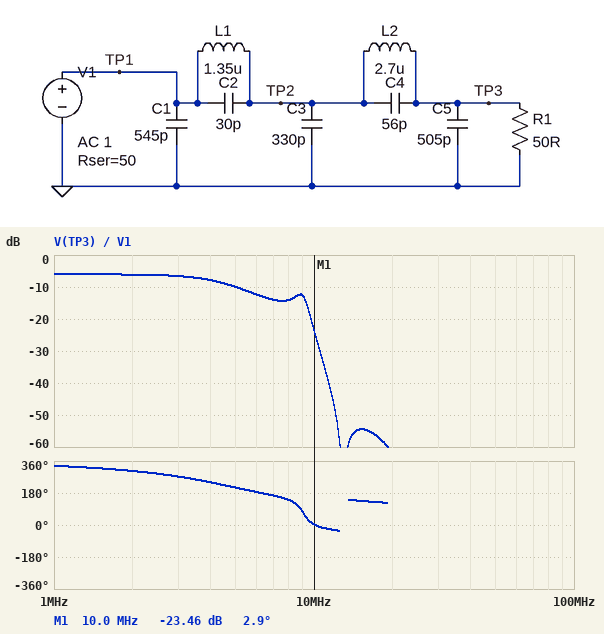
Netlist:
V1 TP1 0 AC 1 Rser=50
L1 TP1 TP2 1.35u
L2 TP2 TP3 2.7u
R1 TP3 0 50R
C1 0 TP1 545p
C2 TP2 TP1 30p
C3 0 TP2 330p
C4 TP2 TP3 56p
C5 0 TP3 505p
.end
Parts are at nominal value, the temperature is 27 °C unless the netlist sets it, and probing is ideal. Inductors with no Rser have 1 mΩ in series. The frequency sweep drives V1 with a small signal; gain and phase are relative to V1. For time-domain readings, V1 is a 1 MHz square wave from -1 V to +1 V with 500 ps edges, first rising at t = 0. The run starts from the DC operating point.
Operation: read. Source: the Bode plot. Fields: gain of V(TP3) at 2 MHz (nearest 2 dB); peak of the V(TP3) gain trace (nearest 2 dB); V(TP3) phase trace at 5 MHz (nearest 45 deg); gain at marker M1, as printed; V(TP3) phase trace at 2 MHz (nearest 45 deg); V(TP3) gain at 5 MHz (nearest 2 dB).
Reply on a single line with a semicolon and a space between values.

-6 dB; -6 dB; 225 deg; -23.46 dB; 315 deg; -10 dB
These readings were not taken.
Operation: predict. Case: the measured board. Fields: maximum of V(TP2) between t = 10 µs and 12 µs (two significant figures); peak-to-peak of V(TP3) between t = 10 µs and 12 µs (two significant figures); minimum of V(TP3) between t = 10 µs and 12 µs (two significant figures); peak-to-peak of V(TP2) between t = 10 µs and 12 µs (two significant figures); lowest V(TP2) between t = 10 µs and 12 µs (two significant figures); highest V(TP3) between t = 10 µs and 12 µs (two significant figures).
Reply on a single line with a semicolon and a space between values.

1.1 V; 1.1 V; -560 mV; 2.2 V; -1.1 V; 560 mV
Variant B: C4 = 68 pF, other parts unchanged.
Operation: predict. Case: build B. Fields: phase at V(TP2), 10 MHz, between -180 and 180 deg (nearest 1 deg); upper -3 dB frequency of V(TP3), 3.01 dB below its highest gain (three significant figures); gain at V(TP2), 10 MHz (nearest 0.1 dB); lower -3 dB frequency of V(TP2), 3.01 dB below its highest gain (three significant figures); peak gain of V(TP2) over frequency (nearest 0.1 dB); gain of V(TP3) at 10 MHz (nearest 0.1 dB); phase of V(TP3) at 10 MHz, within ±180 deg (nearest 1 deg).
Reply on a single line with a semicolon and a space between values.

146 deg; 4.51 MHz; -1.0 dB; 8.27 MHz; 7.1 dB; -27.9 dB; 0 deg
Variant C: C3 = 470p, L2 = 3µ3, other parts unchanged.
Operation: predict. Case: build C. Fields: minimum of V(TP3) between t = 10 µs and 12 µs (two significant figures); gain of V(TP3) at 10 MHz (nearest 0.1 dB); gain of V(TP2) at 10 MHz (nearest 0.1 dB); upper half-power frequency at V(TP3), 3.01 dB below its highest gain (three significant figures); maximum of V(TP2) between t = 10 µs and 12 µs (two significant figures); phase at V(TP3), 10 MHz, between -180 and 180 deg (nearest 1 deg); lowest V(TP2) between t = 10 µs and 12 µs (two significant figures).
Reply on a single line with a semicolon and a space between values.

-540 mV; -37.0 dB; -8.1 dB; 4.16 MHz; 1.0 V; -10 deg; -1.0 V
